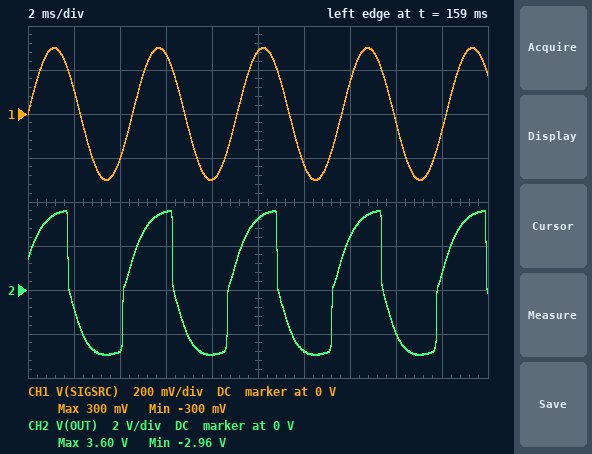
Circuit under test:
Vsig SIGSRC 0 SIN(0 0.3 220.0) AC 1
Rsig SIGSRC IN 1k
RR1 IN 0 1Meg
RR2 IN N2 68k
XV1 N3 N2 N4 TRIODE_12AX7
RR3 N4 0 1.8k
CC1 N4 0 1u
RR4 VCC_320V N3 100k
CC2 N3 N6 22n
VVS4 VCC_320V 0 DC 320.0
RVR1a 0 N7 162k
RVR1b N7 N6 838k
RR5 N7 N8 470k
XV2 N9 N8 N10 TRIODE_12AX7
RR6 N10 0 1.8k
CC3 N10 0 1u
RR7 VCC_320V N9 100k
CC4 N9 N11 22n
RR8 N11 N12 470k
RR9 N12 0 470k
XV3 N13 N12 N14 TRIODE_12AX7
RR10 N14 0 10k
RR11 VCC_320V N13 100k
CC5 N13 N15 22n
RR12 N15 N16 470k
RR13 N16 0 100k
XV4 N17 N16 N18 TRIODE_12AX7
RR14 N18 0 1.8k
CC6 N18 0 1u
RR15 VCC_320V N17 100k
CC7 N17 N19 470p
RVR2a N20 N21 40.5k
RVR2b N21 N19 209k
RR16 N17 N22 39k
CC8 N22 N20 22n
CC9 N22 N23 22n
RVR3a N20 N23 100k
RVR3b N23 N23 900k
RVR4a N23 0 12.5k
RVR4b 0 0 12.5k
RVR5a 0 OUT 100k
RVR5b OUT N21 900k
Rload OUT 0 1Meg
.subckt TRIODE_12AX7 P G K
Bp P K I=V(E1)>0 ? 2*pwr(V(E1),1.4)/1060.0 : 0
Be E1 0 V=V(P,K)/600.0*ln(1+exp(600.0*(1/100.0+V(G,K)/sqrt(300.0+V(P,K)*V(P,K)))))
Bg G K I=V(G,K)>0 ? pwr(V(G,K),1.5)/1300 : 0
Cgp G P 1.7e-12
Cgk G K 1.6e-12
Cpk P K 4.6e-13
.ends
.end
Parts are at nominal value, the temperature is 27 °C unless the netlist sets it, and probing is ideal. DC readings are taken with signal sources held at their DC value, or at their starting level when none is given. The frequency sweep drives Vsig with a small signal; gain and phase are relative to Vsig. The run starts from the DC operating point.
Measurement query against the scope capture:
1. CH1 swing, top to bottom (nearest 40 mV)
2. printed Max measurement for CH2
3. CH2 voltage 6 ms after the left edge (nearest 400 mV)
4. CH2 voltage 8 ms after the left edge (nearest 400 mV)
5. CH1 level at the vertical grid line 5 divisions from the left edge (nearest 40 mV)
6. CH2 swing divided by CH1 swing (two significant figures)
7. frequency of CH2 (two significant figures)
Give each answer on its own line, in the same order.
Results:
600 mV
3.60 V
3.6 V
-2.8 V
280 mV
11
220 Hz
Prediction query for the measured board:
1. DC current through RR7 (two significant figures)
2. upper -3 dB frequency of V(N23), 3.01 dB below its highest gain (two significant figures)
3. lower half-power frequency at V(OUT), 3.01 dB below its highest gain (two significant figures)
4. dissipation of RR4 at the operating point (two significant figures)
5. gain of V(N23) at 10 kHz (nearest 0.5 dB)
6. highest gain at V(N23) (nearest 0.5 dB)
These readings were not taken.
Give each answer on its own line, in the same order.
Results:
950 µA
3.3 kHz
170 Hz
90 mW
56.0 dB
68.0 dB
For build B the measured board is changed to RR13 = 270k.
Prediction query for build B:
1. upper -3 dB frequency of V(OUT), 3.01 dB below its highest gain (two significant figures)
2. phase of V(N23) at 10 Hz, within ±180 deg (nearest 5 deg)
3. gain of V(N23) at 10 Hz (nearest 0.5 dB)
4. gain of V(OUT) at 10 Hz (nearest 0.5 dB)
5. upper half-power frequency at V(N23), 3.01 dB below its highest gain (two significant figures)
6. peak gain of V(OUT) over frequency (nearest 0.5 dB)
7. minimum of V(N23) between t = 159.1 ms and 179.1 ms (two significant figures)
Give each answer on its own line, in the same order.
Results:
2.9 kHz
-170 deg
36.5 dB
29.0 dB
3.2 kHz
57.0 dB
-19 V
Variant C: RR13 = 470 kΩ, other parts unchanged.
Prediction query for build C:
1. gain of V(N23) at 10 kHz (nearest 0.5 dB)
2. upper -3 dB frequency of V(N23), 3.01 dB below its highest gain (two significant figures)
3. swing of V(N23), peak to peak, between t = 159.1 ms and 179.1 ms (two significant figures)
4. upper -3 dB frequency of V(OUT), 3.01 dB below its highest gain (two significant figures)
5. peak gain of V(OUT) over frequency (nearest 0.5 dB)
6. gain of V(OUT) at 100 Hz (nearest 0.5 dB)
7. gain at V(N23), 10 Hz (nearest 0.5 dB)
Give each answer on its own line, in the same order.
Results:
63.0 dB
3.1 kHz
35 V
2.8 kHz
60.0 dB
52.5 dB
40.0 dB
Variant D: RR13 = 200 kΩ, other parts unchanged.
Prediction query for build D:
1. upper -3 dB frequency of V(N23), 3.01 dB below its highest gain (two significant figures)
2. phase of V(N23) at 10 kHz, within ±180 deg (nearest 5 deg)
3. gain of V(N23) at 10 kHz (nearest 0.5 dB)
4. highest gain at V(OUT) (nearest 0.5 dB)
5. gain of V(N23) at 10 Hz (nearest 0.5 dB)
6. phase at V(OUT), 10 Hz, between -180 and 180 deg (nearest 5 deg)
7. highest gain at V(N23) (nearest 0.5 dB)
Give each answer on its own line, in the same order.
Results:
3.2 kHz
-140 deg
60.0 dB
55.0 dB
34.0 dB
-170 deg
73.0 dB
